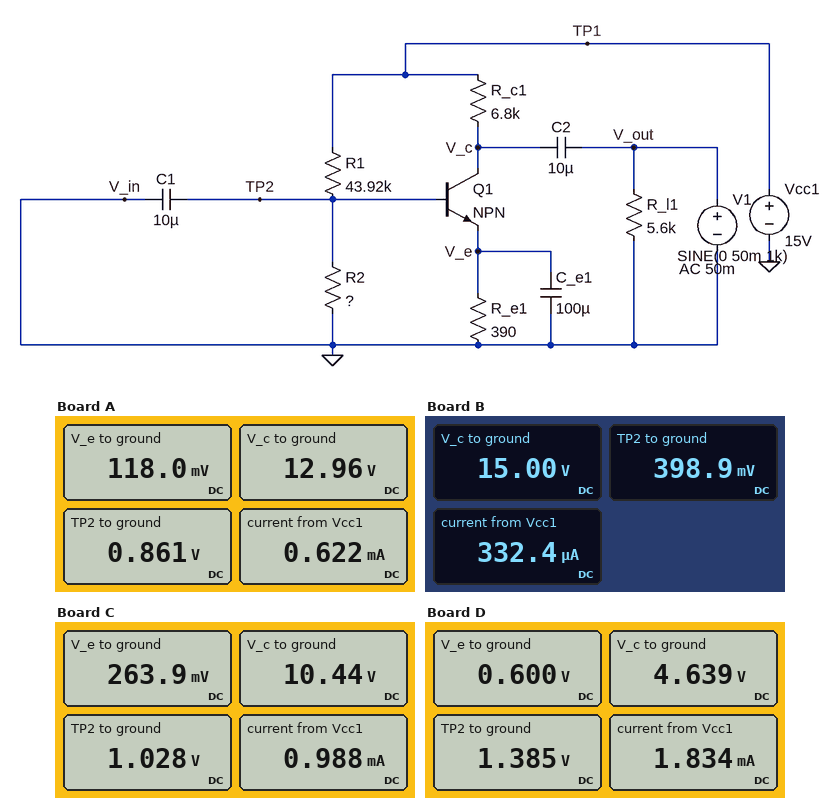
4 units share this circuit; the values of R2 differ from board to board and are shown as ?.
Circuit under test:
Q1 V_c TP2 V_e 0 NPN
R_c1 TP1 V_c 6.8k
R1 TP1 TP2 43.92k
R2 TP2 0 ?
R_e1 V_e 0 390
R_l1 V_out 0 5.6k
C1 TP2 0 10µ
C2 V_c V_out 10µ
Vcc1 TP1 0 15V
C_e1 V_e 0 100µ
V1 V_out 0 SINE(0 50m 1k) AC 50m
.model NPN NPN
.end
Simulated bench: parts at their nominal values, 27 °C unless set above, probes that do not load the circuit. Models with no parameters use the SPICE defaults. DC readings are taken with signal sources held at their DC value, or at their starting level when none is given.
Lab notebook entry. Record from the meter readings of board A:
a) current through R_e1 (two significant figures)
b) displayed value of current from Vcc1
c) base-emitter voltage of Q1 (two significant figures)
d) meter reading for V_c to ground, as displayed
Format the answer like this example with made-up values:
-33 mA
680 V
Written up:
300 µA
0.622 mA
740 mV
12.96 V
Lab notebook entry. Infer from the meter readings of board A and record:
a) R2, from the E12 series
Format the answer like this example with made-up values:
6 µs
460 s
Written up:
2.7 kΩ
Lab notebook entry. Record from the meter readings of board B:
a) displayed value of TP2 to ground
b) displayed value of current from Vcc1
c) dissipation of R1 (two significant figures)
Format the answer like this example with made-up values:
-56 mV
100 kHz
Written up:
398.9 mV
332.4 µA
4.9 mW
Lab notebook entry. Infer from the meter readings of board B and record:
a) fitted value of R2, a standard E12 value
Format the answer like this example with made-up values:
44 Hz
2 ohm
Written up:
1.2 kΩ
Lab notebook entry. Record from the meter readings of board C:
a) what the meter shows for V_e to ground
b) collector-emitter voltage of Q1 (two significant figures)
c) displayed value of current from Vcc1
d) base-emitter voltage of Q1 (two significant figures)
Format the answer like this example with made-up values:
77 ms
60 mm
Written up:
263.9 mV
10 V
0.988 mA
760 mV
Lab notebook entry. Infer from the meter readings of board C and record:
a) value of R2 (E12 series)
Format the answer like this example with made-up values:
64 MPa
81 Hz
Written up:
3.3 kΩ
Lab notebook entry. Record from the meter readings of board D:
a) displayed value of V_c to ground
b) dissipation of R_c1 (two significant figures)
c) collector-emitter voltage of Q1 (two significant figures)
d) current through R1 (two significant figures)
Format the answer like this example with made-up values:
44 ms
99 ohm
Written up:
4.639 V
16 mW
4.0 V
310 µA
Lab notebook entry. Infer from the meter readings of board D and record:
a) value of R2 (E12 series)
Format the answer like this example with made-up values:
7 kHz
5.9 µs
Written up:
4.7 kΩ
